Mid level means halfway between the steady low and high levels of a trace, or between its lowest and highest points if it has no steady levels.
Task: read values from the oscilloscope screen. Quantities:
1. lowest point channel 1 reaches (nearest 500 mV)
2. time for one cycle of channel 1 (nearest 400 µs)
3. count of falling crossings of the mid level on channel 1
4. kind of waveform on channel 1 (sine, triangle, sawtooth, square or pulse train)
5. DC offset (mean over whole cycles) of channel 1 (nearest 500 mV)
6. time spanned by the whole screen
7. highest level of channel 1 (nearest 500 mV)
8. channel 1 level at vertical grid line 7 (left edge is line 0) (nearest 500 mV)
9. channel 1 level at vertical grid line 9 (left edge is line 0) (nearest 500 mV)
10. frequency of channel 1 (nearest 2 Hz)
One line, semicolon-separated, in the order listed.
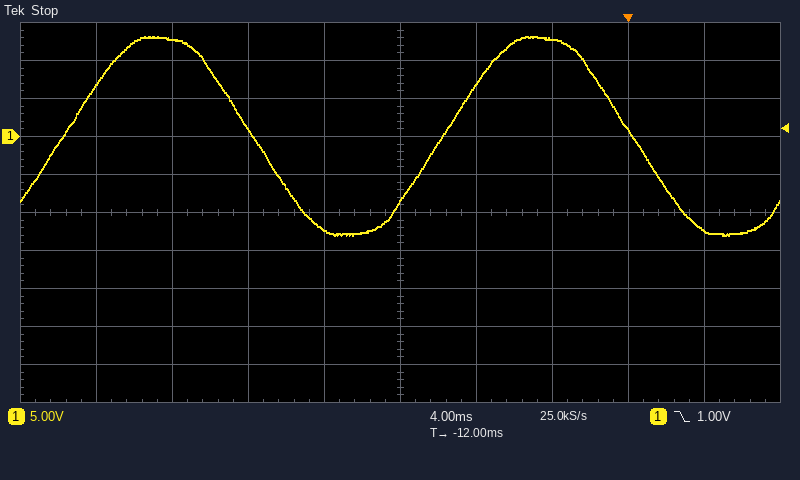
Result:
-13.0 V; 20.0 ms; 2; sine; 0.0 V; 40 ms; 13.0 V; 13.0 V; -12.5 V; 50 Hz
